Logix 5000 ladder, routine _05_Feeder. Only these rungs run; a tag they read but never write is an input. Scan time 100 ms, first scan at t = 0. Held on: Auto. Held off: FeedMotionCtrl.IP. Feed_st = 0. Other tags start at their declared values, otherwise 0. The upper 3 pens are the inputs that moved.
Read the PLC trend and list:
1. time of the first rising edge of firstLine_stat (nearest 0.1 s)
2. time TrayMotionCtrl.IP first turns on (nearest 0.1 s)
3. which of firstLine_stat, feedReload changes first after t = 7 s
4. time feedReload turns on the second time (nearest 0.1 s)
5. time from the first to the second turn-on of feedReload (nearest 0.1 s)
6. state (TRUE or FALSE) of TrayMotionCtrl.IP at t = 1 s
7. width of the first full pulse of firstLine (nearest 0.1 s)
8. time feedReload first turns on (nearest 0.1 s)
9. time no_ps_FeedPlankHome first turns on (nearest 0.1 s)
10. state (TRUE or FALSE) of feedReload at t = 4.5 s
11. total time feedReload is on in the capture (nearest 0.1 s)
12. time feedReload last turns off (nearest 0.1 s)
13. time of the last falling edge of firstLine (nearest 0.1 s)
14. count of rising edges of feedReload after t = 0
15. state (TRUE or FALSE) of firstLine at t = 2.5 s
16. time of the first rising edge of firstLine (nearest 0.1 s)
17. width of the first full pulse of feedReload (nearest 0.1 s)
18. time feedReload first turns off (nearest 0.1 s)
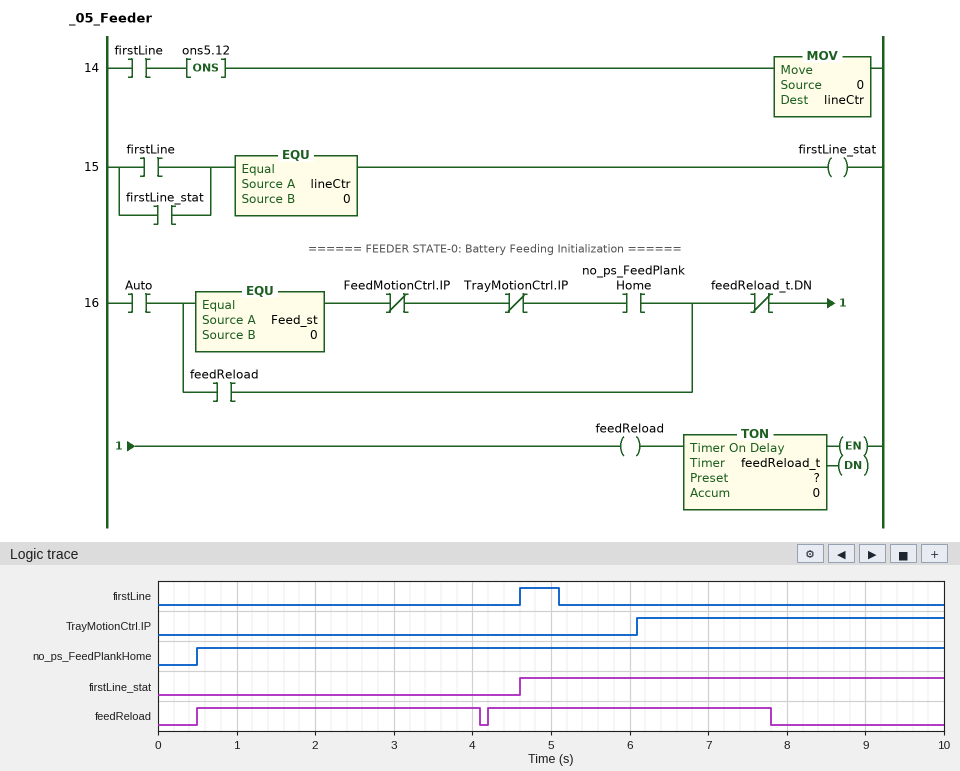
4.6 s
6.1 s
feedReload
4.2 s
3.7 s
FALSE
0.5 s
0.5 s
0.5 s
TRUE
7.2 s
7.8 s
5.1 s
2
FALSE
4.6 s
3.6 s
4.1 s
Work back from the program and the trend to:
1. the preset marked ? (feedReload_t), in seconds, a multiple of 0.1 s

3.5 s
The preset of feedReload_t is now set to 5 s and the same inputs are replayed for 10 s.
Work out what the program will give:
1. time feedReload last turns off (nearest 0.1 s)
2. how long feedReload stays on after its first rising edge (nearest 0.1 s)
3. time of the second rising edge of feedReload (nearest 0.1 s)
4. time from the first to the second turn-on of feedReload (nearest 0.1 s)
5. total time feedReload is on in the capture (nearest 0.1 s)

5.6 s
5.1 s
5.7 s
5.2 s
9.4 s
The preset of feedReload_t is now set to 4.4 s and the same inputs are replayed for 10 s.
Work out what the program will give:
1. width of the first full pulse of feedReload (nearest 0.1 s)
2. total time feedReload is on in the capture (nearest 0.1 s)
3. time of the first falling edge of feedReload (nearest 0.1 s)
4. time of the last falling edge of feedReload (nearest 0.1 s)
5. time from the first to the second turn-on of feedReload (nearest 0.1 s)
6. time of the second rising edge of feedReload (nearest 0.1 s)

4.5 s
9.0 s
5.0 s
9.6 s
4.6 s
5.1 s
